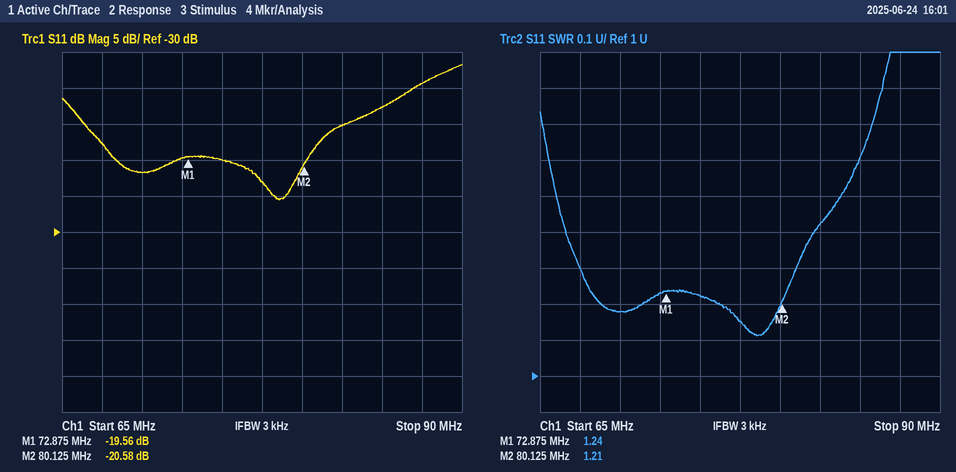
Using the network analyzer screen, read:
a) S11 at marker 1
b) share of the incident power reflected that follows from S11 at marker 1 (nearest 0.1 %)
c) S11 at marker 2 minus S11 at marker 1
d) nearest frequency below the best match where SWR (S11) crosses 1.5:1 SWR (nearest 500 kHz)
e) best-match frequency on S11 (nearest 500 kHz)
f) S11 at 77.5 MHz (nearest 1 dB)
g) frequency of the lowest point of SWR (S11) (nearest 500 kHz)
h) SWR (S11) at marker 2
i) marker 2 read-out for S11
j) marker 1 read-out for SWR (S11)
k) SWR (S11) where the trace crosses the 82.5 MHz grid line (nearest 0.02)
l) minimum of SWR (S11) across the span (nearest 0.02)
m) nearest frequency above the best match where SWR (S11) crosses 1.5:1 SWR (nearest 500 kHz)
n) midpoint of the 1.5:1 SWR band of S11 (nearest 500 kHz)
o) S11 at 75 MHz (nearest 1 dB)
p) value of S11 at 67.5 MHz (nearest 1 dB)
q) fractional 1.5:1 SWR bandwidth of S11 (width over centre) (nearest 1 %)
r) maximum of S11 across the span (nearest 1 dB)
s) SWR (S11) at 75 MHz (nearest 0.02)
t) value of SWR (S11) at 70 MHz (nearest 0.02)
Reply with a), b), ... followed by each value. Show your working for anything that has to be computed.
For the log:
a) -19.56 dB
b) 10^(-19.56/10) ≈ 1.1 %
c) -20.58 − (-19.56) = -1.02 dB
d) 66.0 MHz
e) 78.5 MHz
f) -23 dB
g) 78.5 MHz
h) 1.21
i) -20.58 dB
j) 1.24
k) 1.42
l) 1.12
m) 84.0 MHz
n) 75.0 MHz
o) -20 dB
p) -18 dB
q) 18 MHz / 75 MHz ≈ 24 %
r) -7 dB
s) 1.22
t) 1.18
